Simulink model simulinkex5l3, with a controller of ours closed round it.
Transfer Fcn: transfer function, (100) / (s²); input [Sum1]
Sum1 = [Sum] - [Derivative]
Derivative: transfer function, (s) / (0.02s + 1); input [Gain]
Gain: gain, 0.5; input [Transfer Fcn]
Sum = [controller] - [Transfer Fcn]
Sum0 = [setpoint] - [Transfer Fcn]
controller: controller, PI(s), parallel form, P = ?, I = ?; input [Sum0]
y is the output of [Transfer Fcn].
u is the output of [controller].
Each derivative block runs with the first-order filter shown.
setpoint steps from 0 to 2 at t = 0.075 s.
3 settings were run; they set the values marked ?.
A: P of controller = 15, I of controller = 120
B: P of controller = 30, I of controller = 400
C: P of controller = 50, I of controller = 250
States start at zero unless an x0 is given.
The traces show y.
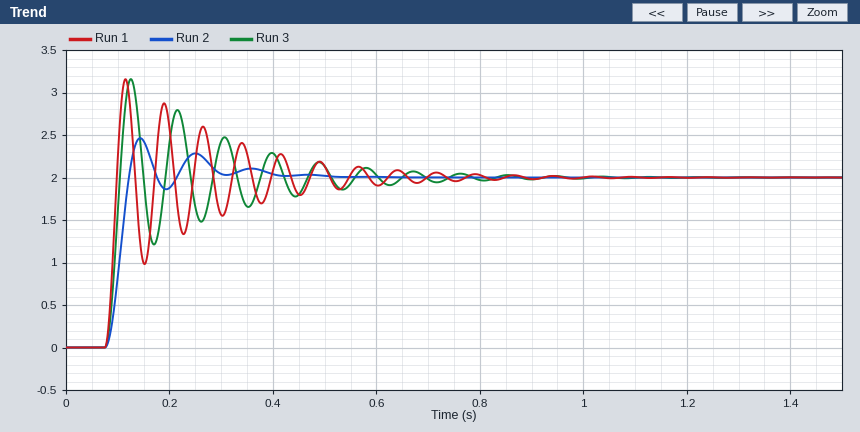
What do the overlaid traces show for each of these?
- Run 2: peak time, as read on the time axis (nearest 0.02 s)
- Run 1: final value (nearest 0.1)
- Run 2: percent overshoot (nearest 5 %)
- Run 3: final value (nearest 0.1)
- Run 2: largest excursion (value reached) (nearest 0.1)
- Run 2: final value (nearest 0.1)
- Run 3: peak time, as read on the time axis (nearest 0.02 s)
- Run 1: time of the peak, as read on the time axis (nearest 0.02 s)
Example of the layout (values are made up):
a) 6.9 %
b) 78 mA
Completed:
a) 0.14 s
b) 2.0
c) 25 %
d) 2.0
e) 2.5
f) 2.0
g) 0.12 s
h) 0.12 s
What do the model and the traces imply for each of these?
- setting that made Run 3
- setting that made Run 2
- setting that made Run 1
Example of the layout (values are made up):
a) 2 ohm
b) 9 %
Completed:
a) B
b) A
c) C
